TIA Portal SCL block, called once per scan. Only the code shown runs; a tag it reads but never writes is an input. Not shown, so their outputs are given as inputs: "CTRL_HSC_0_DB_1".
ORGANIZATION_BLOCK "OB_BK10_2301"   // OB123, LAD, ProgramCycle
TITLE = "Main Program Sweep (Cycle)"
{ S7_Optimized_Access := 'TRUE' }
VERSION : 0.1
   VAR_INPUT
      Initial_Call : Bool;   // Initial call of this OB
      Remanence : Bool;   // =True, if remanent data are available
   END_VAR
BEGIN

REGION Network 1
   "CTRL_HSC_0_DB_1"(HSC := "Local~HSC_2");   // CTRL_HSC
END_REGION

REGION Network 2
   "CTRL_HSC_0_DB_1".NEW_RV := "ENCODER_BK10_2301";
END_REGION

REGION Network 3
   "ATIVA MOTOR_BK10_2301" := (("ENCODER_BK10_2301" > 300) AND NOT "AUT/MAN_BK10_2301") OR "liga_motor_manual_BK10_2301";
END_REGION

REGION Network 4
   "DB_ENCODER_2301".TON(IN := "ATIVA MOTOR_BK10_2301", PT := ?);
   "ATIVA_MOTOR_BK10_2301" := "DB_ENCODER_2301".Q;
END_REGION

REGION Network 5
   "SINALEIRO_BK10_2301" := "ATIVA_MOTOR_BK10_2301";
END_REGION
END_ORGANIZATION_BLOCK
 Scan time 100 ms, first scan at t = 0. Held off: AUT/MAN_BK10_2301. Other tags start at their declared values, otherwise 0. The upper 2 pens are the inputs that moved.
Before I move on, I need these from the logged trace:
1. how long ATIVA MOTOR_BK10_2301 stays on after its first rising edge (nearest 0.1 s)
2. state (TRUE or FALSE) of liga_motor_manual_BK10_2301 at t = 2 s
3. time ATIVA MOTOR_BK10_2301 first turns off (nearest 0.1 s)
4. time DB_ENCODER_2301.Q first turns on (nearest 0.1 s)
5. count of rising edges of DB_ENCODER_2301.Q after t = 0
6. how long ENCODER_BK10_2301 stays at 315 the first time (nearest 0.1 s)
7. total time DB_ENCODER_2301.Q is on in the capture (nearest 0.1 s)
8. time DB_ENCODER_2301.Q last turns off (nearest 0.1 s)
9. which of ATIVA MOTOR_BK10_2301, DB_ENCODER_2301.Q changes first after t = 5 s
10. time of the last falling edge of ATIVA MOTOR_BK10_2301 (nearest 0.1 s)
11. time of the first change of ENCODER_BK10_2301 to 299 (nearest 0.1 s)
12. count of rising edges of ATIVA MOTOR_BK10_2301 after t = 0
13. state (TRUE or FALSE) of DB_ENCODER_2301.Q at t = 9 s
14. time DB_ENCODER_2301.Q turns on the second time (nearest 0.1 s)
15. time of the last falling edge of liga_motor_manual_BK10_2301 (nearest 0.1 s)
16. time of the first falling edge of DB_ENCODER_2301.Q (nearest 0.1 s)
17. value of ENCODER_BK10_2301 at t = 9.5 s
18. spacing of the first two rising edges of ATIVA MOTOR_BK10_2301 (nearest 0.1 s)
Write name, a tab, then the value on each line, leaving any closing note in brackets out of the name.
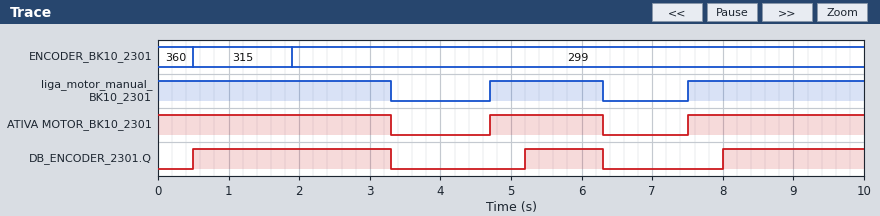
how long ATIVA MOTOR_BK10_2301 stays on after its first rising edge	1.6 s
state (TRUE or FALSE) of liga_motor_manual_BK10_2301 at t = 2 s	TRUE
time ATIVA MOTOR_BK10_2301 first turns off	3.3 s
time DB_ENCODER_2301.Q first turns on	0.5 s
count of rising edges of DB_ENCODER_2301.Q after t = 0	3
how long ENCODER_BK10_2301 stays at 315 the first time	1.4 s
total time DB_ENCODER_2301.Q is on in the capture	5.9 s
time DB_ENCODER_2301.Q last turns off	6.3 s
which of ATIVA MOTOR_BK10_2301, DB_ENCODER_2301.Q changes first after t = 5 s	DB_ENCODER_2301.Q
time of the last falling edge of ATIVA MOTOR_BK10_2301	6.3 s
time of the first change of ENCODER_BK10_2301 to 299	1.9 s
count of rising edges of ATIVA MOTOR_BK10_2301 after t = 0	2
state (TRUE or FALSE) of DB_ENCODER_2301.Q at t = 9 s	TRUE
time DB_ENCODER_2301.Q turns on the second time	5.2 s
time of the last falling edge of liga_motor_manual_BK10_2301	6.3 s
time of the first falling edge of DB_ENCODER_2301.Q	3.3 s
value of ENCODER_BK10_2301 at t = 9.5 s	299
spacing of the first two rising edges of ATIVA MOTOR_BK10_2301	2.8 s
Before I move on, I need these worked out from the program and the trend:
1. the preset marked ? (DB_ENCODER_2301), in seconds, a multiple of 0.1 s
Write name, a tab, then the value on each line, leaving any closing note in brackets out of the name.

the preset marked ? (DB_ENCODER_2301), in seconds, a multiple of 0.1 s	0.5 s
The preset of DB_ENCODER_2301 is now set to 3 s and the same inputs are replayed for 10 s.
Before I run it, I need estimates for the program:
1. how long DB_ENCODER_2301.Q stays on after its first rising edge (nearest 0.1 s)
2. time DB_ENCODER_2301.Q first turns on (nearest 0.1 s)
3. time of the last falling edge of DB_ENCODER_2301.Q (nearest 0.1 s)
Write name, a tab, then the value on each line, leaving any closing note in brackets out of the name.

how long DB_ENCODER_2301.Q stays on after its first rising edge	0.3 s
time DB_ENCODER_2301.Q first turns on	3.0 s
time of the last falling edge of DB_ENCODER_2301.Q	3.3 s
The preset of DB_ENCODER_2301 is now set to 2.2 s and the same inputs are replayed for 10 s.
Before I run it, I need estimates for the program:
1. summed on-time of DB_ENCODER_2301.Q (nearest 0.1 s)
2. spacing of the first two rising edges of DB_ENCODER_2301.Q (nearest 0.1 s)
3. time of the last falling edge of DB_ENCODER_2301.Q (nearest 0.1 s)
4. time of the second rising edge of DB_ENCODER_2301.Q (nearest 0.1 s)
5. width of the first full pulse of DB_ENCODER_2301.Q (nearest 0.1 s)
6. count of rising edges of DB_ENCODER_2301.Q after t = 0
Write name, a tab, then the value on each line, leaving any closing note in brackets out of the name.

summed on-time of DB_ENCODER_2301.Q	1.4 s
spacing of the first two rising edges of DB_ENCODER_2301.Q	7.5 s
time of the last falling edge of DB_ENCODER_2301.Q	3.3 s
time of the second rising edge of DB_ENCODER_2301.Q	9.7 s
width of the first full pulse of DB_ENCODER_2301.Q	1.1 s
count of rising edges of DB_ENCODER_2301.Q after t = 0	2
